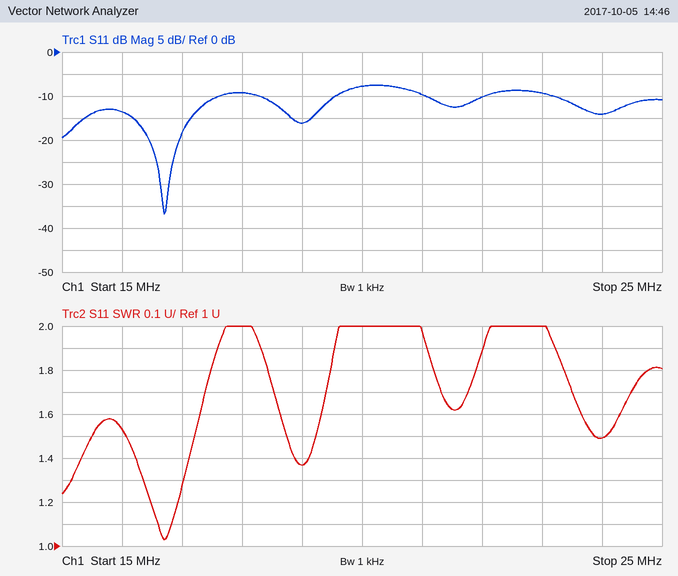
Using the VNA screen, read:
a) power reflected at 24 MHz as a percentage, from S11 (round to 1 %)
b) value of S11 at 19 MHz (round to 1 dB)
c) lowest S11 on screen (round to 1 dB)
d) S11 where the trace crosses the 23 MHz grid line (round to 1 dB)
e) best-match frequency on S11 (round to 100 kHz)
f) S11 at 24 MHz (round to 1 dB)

4 %
-16 dB
-37 dB
-9 dB
16.7 MHz
-14 dB
